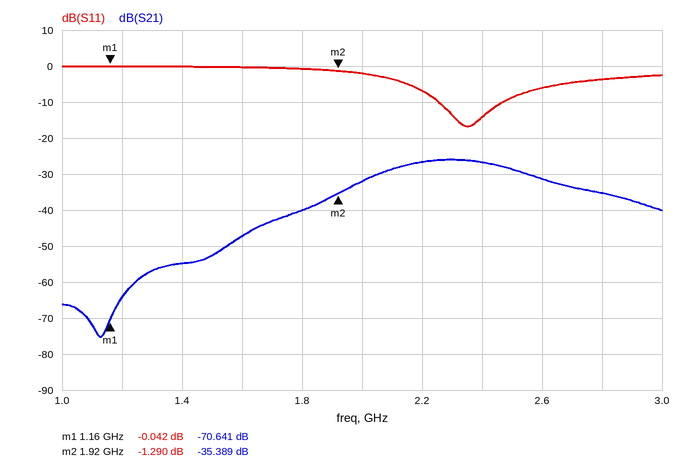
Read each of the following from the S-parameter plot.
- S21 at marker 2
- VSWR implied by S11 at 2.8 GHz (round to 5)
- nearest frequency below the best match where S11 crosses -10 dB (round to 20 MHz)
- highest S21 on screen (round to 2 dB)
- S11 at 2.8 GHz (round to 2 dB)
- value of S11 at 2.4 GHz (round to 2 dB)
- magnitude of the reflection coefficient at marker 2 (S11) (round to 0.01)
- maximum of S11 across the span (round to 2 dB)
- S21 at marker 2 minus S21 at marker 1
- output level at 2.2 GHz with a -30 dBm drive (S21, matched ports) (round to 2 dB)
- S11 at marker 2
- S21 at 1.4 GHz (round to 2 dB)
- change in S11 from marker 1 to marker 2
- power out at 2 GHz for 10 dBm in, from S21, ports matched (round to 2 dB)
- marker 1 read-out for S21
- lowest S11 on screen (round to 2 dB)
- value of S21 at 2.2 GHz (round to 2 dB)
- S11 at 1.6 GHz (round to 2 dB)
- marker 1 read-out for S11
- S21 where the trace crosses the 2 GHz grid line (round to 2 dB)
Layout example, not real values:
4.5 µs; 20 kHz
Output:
-35.389 dB; 5; 2.26 GHz; -26 dB; -4 dB; -14 dB; 0.86; 0 dB; 35.252 dB; -56 dBm; -1.290 dB; -54 dB; -1.248 dB; -22 dBm; -70.641 dB; -16 dB; -26 dB; 0 dB; -0.042 dB; -32 dB
